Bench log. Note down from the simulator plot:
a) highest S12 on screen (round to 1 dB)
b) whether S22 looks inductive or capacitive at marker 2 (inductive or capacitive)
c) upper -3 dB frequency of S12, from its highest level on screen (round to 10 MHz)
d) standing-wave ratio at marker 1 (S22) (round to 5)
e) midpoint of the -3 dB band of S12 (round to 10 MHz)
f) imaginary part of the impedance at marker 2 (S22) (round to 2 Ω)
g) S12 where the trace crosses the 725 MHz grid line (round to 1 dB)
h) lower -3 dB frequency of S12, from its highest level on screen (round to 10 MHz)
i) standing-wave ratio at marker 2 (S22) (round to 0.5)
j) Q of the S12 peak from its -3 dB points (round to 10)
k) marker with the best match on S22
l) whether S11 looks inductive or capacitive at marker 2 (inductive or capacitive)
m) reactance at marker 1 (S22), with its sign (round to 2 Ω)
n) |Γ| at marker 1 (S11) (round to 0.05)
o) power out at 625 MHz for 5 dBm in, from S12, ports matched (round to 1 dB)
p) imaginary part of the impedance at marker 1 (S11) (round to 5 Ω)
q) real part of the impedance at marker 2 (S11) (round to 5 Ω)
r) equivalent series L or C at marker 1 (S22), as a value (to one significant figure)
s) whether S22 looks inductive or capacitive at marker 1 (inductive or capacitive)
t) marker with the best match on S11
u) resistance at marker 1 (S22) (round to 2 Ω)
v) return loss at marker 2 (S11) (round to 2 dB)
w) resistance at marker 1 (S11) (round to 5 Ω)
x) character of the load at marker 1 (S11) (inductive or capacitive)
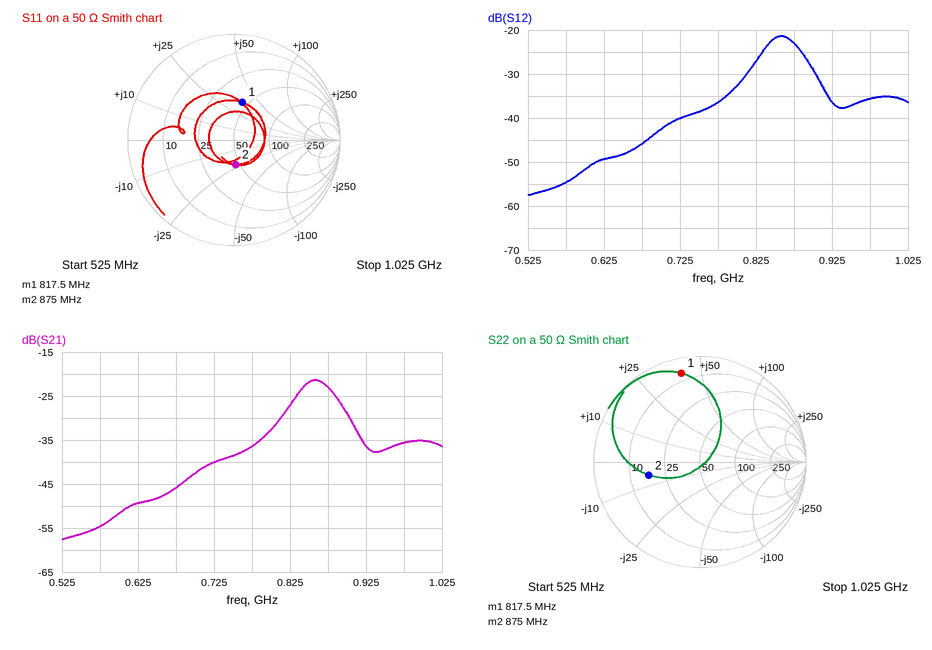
-21 dB
capacitive
880 MHz
15
860 MHz
-6 Ω
-40 dB
840 MHz
3.0
20
marker 2
capacitive
+40 Ω
0.35
-44 dBm
+35 Ω
45 Ω
8 nH
inductive
marker 2
6 Ω
12 dB
45 Ω
inductive
